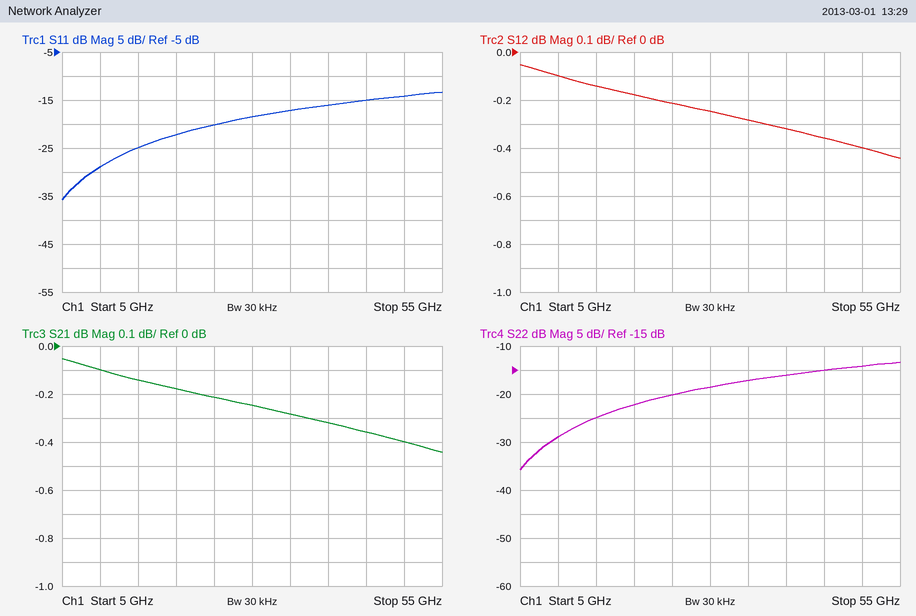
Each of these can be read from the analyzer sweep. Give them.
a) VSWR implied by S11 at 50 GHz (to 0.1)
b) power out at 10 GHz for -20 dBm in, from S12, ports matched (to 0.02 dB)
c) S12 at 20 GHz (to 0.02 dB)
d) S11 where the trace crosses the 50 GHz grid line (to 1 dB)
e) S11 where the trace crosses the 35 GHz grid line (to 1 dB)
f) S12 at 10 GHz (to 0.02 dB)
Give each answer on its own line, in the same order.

1.5
-20.10 dBm
-0.18 dB
-14 dB
-17 dB
-0.10 dB
